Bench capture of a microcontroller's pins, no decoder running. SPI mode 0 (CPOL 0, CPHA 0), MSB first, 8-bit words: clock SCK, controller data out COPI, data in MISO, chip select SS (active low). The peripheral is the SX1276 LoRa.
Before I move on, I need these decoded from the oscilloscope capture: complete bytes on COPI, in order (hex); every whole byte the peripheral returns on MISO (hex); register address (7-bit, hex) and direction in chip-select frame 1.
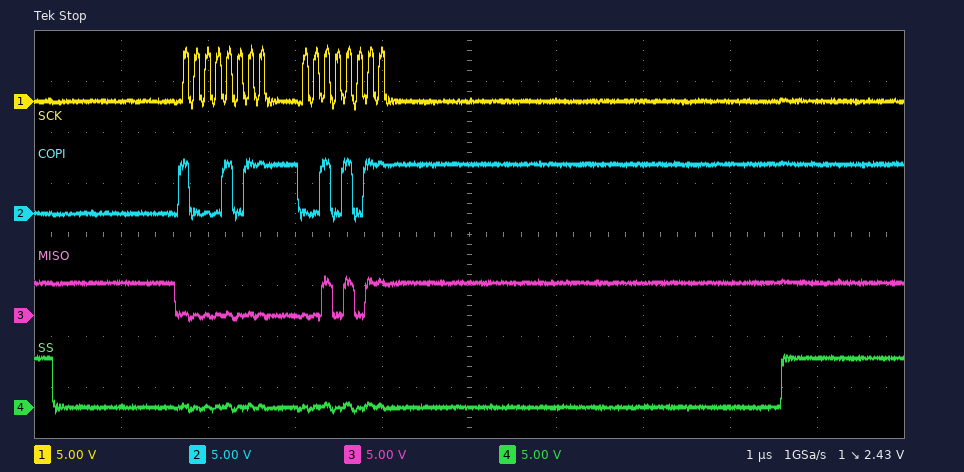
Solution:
0x8B 0x2B
0x00 0x2B
0x0B write
